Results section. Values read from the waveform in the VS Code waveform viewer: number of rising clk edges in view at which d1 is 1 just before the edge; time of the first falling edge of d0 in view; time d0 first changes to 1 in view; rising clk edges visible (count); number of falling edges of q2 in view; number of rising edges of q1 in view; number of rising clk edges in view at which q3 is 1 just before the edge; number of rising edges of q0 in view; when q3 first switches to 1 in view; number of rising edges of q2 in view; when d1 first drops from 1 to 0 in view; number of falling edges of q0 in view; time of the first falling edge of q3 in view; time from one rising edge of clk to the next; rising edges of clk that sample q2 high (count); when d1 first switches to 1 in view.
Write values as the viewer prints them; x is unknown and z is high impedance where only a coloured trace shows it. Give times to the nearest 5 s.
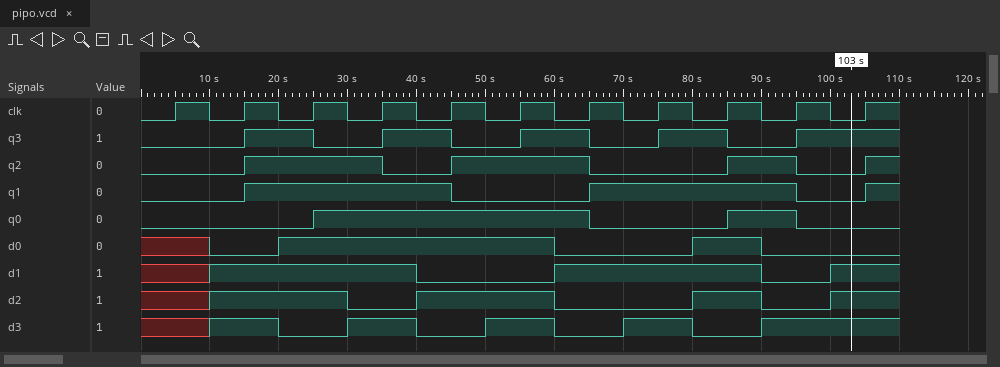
7
60 s
20 s
11
3
3
5
2
15 s
4
40 s
2
25 s
10 s
5
10 s
